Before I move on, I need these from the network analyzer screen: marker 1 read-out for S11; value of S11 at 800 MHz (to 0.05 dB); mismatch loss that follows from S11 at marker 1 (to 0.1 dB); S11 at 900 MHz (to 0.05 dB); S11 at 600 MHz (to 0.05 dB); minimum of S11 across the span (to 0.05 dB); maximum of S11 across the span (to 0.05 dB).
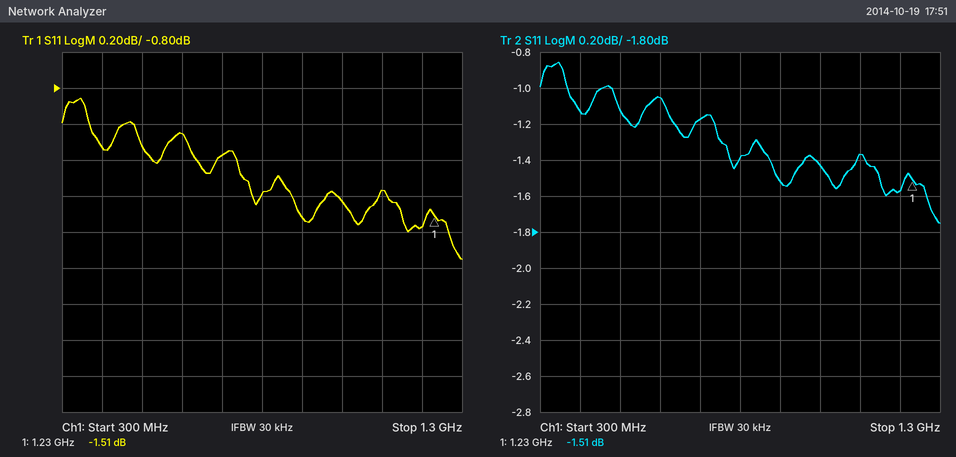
-1.51 dB
-1.40 dB
5.3 dB
-1.50 dB
-1.05 dB
-1.75 dB
-0.85 dB
